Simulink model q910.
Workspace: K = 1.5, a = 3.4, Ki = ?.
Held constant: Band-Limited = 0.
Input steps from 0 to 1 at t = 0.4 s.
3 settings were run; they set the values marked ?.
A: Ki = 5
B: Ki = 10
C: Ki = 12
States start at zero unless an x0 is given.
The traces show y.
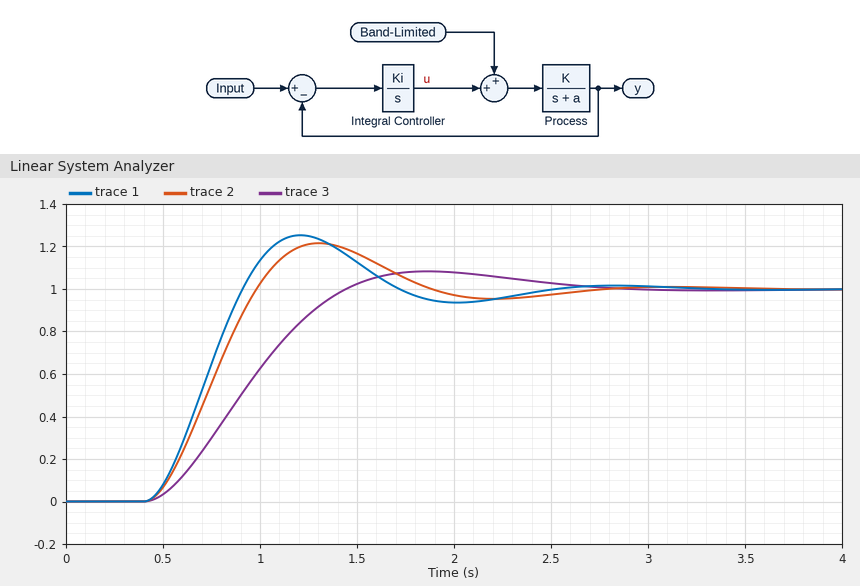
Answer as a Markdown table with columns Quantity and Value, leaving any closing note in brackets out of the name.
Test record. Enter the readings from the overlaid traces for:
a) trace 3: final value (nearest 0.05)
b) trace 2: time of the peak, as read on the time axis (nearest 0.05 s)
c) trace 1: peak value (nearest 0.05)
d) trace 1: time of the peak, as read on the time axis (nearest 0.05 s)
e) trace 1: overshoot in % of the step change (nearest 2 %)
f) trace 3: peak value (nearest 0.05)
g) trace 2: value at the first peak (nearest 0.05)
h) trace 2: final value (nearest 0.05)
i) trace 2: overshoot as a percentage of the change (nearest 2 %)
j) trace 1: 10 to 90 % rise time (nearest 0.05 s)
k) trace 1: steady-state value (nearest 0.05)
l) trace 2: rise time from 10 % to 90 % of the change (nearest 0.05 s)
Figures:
| Quantity | Value |
|---|---|
| trace 3: final value | 1.00 |
| trace 2: time of the peak, as read on the time axis | 1.30 s |
| trace 1: peak value | 1.25 |
| trace 1: time of the peak, as read on the time axis | 1.20 s |
| trace 1: overshoot in % of the step change | 26 % |
| trace 3: peak value | 1.10 |
| trace 2: value at the first peak | 1.20 |
| trace 2: final value | 1.00 |
| trace 2: overshoot as a percentage of the change | 22 % |
| trace 1: 10 to 90 % rise time | 0.35 s |
| trace 1: steady-state value | 1.00 |
| trace 2: rise time from 10 % to 90 % of the change | 0.40 s |
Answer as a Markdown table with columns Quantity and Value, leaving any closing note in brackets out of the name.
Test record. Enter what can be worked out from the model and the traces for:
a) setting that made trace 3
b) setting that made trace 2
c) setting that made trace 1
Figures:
| Quantity | Value |
|---|---|
| setting that made trace 3 | A |
| setting that made trace 2 | B |
| setting that made trace 1 | C |
